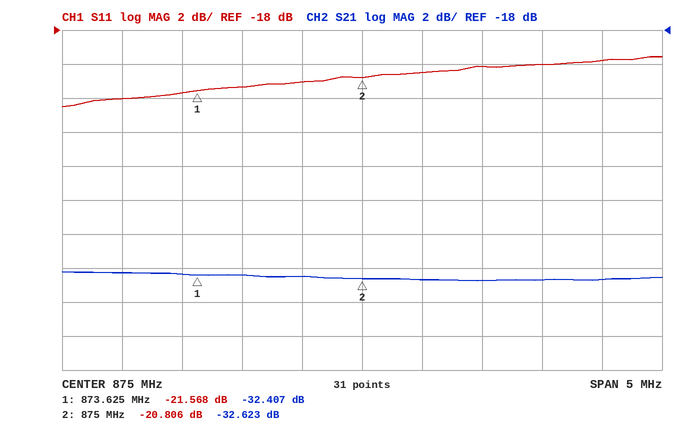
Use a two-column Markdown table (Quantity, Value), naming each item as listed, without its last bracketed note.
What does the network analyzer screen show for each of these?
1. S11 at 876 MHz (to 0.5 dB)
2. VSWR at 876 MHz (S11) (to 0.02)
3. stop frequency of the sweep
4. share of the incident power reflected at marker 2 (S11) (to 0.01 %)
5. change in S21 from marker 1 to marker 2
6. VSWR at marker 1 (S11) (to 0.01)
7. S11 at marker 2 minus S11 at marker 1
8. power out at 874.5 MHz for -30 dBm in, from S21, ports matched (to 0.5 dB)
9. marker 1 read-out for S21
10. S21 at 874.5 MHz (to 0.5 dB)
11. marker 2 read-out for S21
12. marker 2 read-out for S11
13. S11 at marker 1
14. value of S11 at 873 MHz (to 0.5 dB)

| Quantity | Value |
|---|---|
| S11 at 876 MHz | -20.0 dB |
| VSWR at 876 MHz (S11) | 1.22 |
| stop frequency of the sweep | 877.5 MHz |
| share of the incident power reflected at marker 2 (S11) | 0.83 % |
| change in S21 from marker 1 to marker 2 | -0.216 dB |
| VSWR at marker 1 (S11) | 1.18 |
| S11 at marker 2 minus S11 at marker 1 | 0.762 dB |
| power out at 874.5 MHz for -30 dBm in, from S21, ports matched | -62.5 dBm |
| marker 1 read-out for S21 | -32.407 dB |
| S21 at 874.5 MHz | -32.5 dB |
| marker 2 read-out for S21 | -32.623 dB |
| marker 2 read-out for S11 | -20.806 dB |
| S11 at marker 1 | -21.568 dB |
| value of S11 at 873 MHz | -22.0 dB |
